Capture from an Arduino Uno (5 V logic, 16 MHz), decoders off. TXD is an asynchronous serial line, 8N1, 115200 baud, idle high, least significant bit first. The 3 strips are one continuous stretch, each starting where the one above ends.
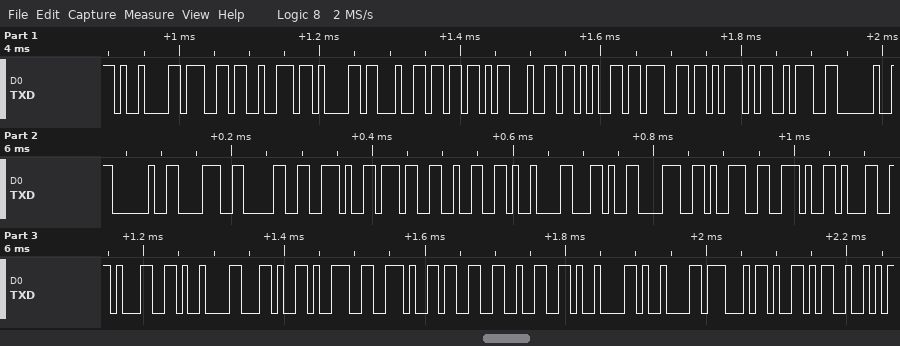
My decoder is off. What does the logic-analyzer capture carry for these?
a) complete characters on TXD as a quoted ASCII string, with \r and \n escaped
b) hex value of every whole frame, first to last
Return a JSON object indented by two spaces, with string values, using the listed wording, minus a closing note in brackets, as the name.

{
  "complete characters on TXD as a quoted ASCII string, with \\r and \\n escaped": "\"\\tgrad[deg]:  80.72\\t,89.11\\t,9.32\\t\\tGYR\"",
  "hex value of every whole frame, first to last": "09 67 72 61 64 5B 64 65 67 5D 3A 20 20 38 30 2E 37 32 09 2C 38 39 2E 31 31 09 2C 39 2E 33 32 09 09 47 59 52"
}
